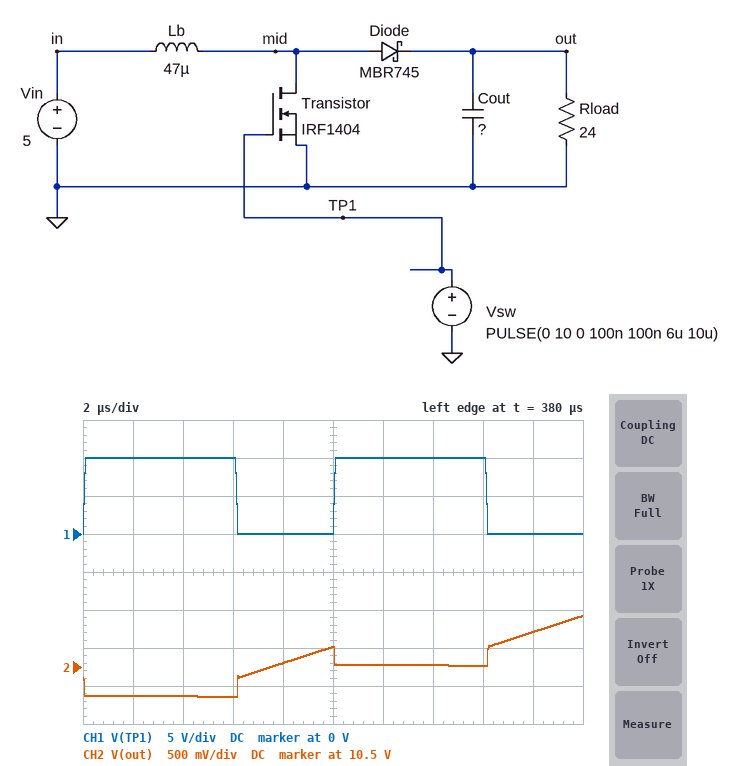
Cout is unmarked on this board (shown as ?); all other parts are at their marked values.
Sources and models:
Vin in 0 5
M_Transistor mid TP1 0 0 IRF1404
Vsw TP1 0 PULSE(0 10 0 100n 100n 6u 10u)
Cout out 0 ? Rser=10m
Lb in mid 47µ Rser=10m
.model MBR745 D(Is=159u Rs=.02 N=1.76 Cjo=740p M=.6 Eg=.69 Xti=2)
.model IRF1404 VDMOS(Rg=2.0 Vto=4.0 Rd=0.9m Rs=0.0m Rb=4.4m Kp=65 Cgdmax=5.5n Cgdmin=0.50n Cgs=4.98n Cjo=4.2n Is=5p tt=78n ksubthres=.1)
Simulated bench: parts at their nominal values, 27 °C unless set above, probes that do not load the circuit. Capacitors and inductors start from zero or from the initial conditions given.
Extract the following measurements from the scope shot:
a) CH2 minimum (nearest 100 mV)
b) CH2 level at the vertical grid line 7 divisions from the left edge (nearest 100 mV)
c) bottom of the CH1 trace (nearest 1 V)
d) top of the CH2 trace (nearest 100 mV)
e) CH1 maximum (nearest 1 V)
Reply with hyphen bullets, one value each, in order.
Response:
- 10.1 V
- 10.5 V
- 0 V
- 11.2 V
- 10 V
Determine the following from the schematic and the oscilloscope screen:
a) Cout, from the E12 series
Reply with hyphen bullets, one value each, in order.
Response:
- 220 µF
